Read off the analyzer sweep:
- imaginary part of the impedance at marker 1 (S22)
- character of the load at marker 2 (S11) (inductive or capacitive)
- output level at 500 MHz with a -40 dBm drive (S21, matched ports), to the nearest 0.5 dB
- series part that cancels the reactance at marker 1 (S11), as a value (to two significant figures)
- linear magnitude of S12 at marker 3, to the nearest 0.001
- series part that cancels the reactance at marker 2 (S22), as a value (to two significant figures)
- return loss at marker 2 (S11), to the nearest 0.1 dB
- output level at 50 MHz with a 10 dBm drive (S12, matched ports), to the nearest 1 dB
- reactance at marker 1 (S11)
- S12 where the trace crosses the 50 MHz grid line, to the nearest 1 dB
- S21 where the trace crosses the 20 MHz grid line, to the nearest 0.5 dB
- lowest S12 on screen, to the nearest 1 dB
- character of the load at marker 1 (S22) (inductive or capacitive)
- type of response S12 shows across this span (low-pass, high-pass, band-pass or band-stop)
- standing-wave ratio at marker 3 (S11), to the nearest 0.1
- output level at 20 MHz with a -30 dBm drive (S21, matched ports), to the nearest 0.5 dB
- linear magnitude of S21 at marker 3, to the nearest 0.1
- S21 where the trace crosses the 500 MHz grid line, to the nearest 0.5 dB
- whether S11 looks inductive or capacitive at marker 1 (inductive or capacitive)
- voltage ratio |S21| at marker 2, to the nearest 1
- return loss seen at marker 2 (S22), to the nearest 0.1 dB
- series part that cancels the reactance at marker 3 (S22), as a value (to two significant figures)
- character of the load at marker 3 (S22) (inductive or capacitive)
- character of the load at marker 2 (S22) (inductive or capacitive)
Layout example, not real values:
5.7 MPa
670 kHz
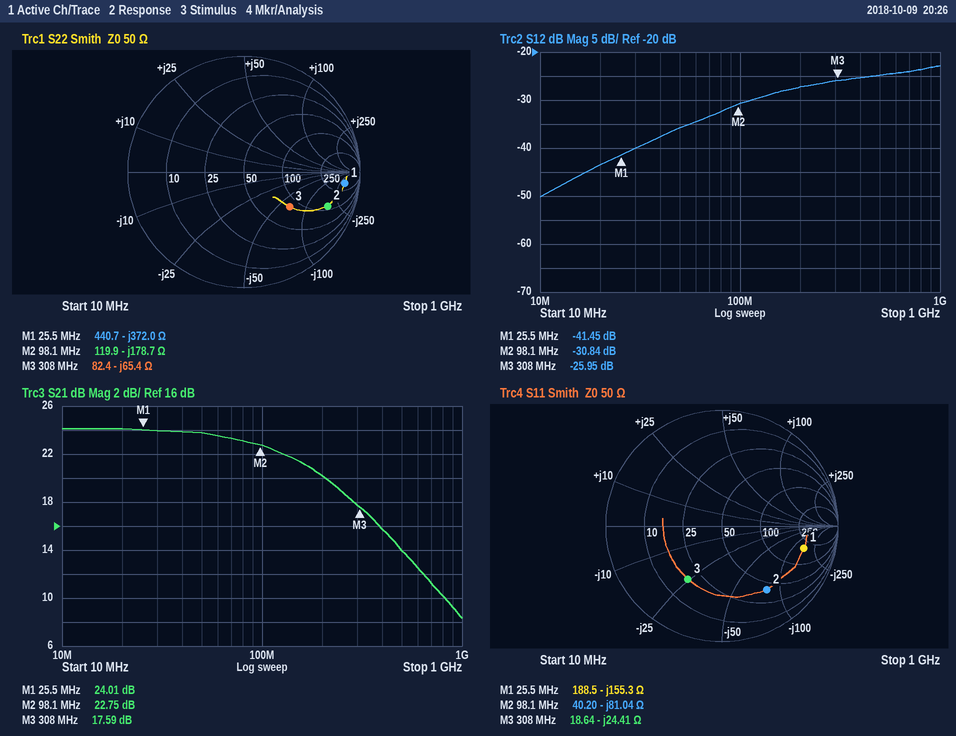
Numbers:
-372.0 Ω
capacitive
-26.0 dBm
970 nH
0.050
290 nH
3.4 dB
-26 dBm
-155.3 Ω
-36 dB
24.0 dB
-50 dB
capacitive
high-pass
3.4
-6.0 dBm
7.6
14.0 dB
capacitive
14
2.2 dB
34 nH
capacitive
capacitive
